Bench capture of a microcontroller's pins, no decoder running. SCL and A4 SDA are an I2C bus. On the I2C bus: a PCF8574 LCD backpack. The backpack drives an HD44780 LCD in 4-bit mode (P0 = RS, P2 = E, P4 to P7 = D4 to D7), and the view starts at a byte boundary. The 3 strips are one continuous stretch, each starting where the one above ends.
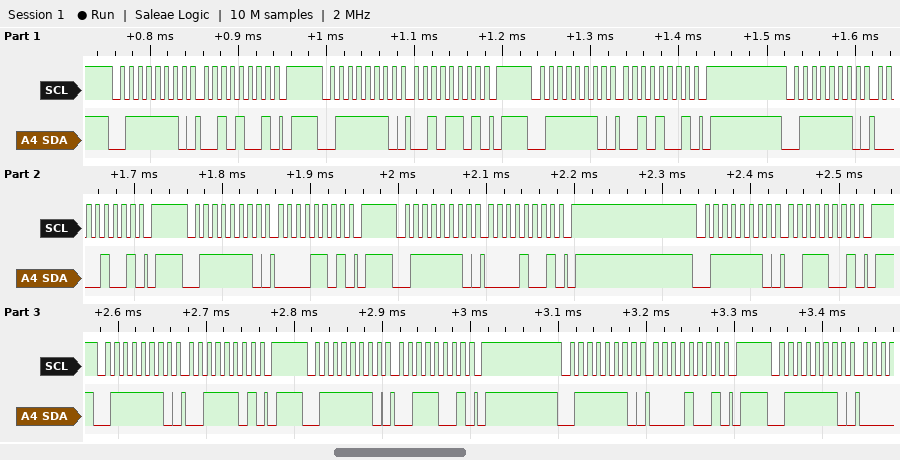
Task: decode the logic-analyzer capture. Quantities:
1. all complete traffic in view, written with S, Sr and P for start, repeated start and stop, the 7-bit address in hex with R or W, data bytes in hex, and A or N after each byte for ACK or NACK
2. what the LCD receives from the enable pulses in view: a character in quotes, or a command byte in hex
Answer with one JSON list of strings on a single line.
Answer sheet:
["S 3FW A 29 A P S 3FW A 2D A P S 3FW A 29 A P S 3FW A 09 A P S 3FW A 0D A P S 3FW A 09 A P S 3FW A 39 A P S 3FW A 3D A P S 3FW A 39 A P S 3FW A 09 A P S 3FW A", "' '"]
